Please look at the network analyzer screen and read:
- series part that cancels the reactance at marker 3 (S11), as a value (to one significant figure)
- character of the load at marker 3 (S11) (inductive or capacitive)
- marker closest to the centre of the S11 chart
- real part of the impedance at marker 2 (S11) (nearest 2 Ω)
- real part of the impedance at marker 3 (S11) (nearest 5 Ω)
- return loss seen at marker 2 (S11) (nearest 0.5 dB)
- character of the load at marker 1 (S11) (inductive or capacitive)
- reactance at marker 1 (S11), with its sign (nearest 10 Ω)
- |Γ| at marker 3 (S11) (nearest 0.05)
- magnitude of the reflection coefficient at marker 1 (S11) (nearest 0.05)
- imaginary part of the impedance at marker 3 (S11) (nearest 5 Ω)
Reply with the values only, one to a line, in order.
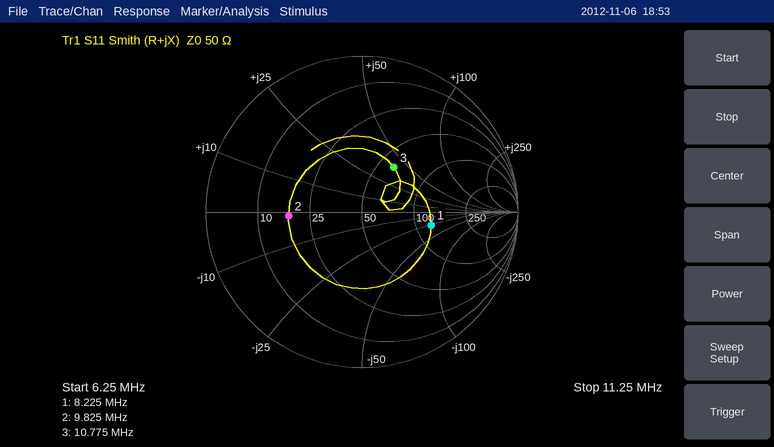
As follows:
400 pF
inductive
marker 3
18 Ω
60 Ω
6.5 dB
capacitive
-30 Ω
0.35
0.45
+40 Ω
